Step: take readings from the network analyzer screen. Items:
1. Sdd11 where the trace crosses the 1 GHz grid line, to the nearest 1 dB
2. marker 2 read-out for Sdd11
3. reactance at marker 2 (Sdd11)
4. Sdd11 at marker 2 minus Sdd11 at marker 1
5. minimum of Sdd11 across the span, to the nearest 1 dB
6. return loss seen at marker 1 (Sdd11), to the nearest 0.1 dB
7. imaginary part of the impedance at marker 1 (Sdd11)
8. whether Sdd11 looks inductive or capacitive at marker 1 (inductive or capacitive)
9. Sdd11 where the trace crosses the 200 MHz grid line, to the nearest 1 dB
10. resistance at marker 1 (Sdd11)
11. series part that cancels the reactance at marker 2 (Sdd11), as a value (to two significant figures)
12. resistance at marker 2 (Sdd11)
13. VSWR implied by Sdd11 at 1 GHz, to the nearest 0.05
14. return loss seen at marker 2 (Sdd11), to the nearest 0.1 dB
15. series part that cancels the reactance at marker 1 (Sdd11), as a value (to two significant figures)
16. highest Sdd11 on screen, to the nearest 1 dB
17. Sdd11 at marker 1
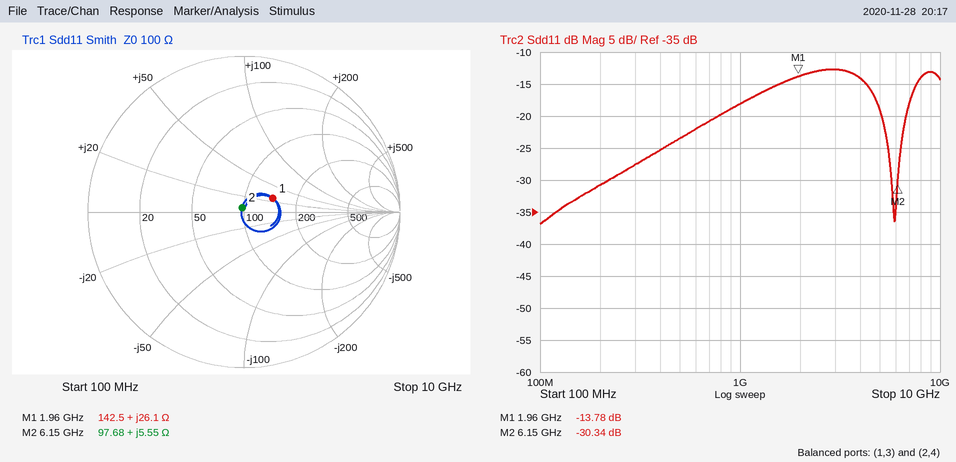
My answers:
-18 dB
-30.34 dB
+5.55 Ω
-16.56 dB
-37 dB
13.8 dB
+26.1 Ω
inductive
-31 dB
142.5 Ω
4.7 pF
97.68 Ω
1.30
30.3 dB
3.1 pF
-13 dB
-13.78 dB
